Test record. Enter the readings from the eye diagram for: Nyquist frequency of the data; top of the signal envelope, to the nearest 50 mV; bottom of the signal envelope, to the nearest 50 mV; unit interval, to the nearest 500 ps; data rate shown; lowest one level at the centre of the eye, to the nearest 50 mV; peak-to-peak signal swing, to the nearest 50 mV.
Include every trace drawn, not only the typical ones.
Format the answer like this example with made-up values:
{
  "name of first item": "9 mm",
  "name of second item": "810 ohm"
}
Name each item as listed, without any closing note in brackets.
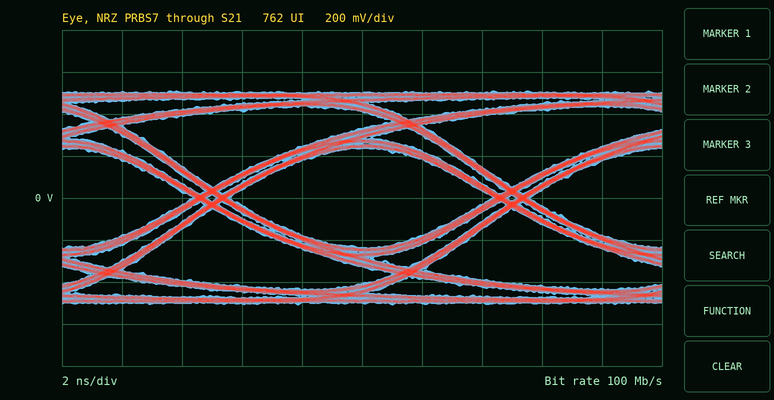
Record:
{
  "Nyquist frequency of the data": "50 MHz",
  "top of the signal envelope, to the nearest 50 mV": "500 mV",
  "bottom of the signal envelope, to the nearest 50 mV": "-500 mV",
  "unit interval, to the nearest 500 ps": "10.0 ns",
  "data rate shown": "100 Mb/s",
  "lowest one level at the centre of the eye, to the nearest 50 mV": "250 mV",
  "peak-to-peak signal swing, to the nearest 50 mV": "1.00 V"
}
